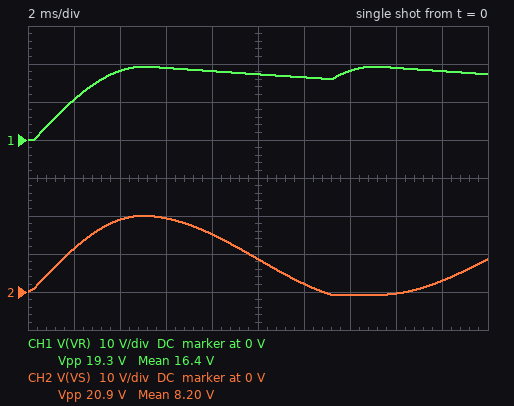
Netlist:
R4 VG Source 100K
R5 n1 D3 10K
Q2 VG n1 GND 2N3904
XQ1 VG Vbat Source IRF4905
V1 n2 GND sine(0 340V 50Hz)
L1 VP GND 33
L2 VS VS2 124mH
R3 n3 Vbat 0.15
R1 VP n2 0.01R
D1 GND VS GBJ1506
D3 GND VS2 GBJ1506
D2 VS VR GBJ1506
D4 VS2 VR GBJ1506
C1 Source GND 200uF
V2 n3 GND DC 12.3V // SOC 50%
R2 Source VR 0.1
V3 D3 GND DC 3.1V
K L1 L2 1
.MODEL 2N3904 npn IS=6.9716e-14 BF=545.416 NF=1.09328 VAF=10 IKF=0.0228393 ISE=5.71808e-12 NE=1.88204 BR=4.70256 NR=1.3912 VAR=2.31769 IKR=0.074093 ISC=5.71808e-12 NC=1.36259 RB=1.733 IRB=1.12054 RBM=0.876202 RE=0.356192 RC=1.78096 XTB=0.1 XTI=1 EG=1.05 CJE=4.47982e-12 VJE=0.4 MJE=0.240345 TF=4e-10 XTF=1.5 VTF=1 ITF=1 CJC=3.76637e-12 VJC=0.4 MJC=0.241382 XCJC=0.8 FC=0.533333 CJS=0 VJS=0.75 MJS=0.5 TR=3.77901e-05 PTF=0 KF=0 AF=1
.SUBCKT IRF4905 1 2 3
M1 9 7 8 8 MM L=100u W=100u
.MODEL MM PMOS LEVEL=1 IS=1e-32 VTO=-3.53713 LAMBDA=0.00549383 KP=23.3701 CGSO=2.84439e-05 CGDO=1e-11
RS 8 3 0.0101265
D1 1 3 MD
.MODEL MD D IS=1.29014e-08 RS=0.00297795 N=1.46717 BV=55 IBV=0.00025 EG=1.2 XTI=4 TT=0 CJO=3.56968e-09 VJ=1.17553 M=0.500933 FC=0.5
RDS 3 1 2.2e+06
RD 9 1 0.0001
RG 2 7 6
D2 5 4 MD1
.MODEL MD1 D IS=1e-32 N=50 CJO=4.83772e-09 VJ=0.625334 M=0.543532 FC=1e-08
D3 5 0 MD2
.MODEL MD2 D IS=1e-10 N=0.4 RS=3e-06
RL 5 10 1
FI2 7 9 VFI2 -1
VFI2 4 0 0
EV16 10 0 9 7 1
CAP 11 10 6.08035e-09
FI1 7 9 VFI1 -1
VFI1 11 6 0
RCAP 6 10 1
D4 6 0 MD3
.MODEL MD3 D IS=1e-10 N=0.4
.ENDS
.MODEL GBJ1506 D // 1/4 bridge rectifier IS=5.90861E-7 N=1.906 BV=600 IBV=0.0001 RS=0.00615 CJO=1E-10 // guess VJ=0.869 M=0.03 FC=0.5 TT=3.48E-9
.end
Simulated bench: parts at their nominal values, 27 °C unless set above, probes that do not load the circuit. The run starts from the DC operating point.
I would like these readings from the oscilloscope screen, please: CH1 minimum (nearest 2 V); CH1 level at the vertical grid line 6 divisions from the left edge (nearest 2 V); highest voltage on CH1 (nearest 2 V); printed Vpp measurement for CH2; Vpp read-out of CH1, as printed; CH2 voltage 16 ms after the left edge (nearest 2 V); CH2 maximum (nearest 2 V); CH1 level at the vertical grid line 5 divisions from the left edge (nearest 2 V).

0 V
16 V
20 V
20.9 V
19.3 V
0 V
20 V
18 V
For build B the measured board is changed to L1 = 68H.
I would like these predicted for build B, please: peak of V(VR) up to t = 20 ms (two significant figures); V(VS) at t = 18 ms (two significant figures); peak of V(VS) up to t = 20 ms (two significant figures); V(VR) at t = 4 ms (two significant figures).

13 V
2.3 V
14 V
12 V
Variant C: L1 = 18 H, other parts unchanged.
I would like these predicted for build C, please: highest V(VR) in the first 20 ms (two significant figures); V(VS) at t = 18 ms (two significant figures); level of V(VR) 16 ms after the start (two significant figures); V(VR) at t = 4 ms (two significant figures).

27 V
4.3 V
26 V
25 V
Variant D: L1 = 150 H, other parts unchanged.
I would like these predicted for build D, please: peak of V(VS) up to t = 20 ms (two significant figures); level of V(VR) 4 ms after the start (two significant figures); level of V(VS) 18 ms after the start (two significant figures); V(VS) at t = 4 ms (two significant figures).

9.0 V
7.7 V
1.3 V
8.5 V
